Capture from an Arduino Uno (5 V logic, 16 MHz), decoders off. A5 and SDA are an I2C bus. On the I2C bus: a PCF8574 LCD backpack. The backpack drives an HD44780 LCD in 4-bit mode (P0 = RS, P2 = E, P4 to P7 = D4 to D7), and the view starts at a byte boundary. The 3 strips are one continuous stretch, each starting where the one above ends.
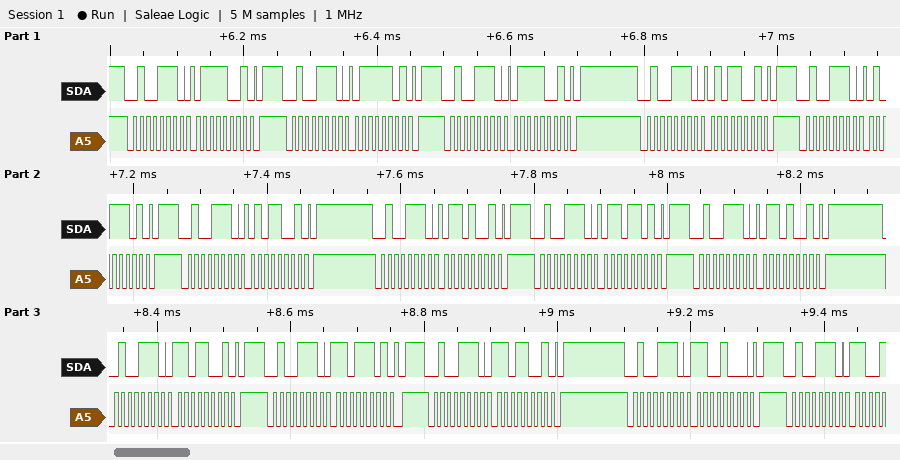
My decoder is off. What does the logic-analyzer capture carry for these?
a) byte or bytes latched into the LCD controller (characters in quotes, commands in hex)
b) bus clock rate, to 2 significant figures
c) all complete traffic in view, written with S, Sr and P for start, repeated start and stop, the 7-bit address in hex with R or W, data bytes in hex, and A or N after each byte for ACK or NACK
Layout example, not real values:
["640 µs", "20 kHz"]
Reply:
["'u' 'm'", "100 kHz", "S 27W A 79 A P S 27W A 7D A P S 27W A 79 A P S 27W A 59 A P S 27W A 5D A P S 27W A 59 A P S 27W A 69 A P S 27W A 6D A P S 27W A 69 A P S 27W A D9 A P S 27W A DD A P S 27W A D9 A P S 27W A C8 A P S 27W A"]
